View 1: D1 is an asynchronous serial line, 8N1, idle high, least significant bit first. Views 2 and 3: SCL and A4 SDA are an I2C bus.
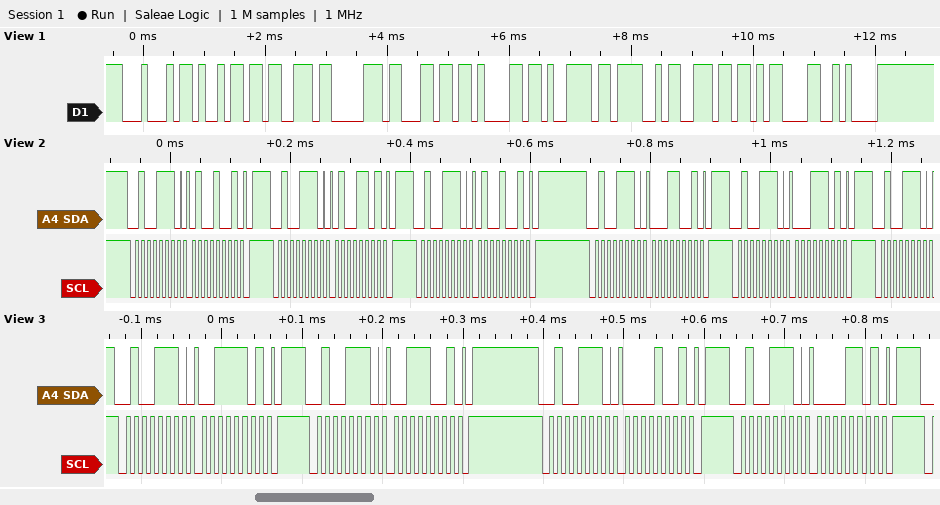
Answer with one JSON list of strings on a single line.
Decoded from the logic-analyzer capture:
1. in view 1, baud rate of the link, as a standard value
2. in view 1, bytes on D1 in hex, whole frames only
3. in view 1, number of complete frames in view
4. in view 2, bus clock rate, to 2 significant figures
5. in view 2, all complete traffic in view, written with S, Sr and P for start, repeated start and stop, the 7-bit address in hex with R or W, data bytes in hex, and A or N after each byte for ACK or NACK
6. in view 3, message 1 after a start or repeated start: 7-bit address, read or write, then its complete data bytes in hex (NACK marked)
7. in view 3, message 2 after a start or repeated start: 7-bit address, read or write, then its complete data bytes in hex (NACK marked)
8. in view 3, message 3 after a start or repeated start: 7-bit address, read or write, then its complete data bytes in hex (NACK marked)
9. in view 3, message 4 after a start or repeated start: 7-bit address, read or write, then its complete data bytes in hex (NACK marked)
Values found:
["9600 baud", "44 69 73 70 6C 61 79 4F 6E 0D 0A", "11", "100 kHz", "S 27W A 49 A P S 27W A 4D A P S 27W A 49 A P S 27W A 19 A P S 27W A 1D A P S 27W A", "0x27 write: 3D", "0x27 write: 39", "0x27 write: 09", "0x27 write: 0D"]
